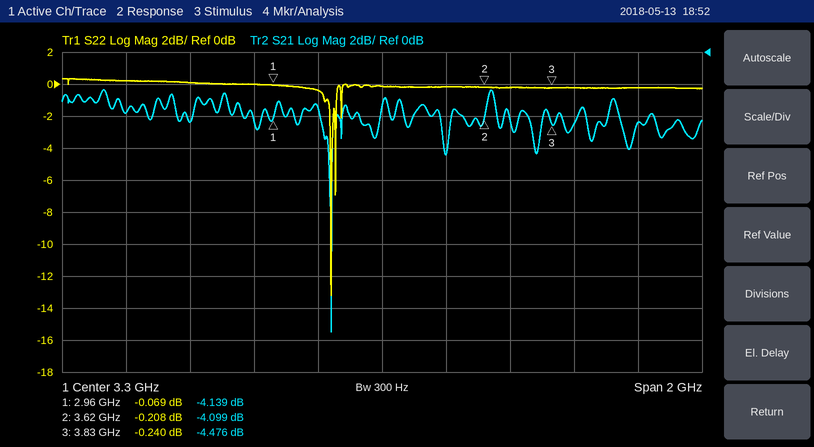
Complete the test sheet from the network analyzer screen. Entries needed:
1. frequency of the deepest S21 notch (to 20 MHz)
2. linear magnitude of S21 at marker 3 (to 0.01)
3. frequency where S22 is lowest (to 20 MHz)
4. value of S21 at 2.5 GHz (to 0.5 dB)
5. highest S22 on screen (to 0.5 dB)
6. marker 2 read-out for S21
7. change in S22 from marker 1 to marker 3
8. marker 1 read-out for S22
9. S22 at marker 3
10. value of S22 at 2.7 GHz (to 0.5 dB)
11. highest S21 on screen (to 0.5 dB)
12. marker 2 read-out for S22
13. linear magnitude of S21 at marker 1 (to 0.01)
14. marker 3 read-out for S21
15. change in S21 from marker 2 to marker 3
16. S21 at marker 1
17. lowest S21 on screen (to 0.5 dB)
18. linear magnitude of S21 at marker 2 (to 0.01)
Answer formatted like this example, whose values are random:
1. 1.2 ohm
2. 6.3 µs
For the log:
1. 3.14 GHz
2. 0.60
3. 3.14 GHz
4. -4.0 dB
5. 0.5 dB
6. -4.099 dB
7. -0.171 dB
8. -0.069 dB
9. -0.240 dB
10. 0.0 dB
11. -2.5 dB
12. -0.208 dB
13. 0.62
14. -4.476 dB
15. -0.377 dB
16. -4.139 dB
17. -17.5 dB
18. 0.62
